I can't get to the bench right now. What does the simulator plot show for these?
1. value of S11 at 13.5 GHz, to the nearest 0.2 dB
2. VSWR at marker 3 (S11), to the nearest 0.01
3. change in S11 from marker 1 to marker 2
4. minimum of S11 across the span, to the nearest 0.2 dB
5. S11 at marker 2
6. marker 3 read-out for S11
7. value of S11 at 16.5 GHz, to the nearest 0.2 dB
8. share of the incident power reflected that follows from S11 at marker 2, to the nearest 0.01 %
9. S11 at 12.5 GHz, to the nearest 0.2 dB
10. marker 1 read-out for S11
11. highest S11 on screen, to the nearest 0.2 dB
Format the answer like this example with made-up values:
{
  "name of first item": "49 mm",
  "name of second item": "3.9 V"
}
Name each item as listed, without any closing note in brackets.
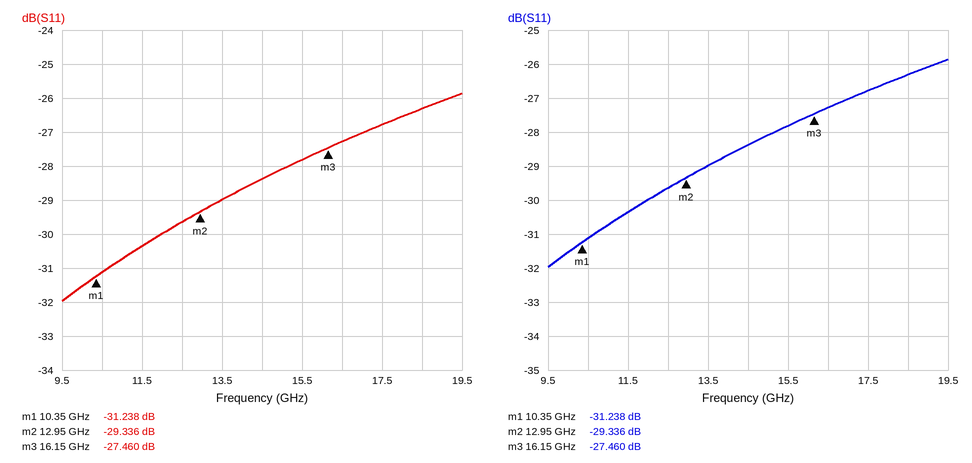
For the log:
{
  "value of S11 at 13.5 GHz, to the nearest 0.2 dB": "-29.0 dB",
  "VSWR at marker 3 (S11), to the nearest 0.01": "1.09",
  "change in S11 from marker 1 to marker 2": "1.902 dB",
  "minimum of S11 across the span, to the nearest 0.2 dB": "-32.0 dB",
  "S11 at marker 2": "-29.336 dB",
  "marker 3 read-out for S11": "-27.460 dB",
  "value of S11 at 16.5 GHz, to the nearest 0.2 dB": "-27.2 dB",
  "share of the incident power reflected that follows from S11 at marker 2, to the nearest 0.01 %": "0.12 %",
  "S11 at 12.5 GHz, to the nearest 0.2 dB": "-29.6 dB",
  "marker 1 read-out for S11": "-31.238 dB",
  "highest S11 on screen, to the nearest 0.2 dB": "-25.8 dB"
}
